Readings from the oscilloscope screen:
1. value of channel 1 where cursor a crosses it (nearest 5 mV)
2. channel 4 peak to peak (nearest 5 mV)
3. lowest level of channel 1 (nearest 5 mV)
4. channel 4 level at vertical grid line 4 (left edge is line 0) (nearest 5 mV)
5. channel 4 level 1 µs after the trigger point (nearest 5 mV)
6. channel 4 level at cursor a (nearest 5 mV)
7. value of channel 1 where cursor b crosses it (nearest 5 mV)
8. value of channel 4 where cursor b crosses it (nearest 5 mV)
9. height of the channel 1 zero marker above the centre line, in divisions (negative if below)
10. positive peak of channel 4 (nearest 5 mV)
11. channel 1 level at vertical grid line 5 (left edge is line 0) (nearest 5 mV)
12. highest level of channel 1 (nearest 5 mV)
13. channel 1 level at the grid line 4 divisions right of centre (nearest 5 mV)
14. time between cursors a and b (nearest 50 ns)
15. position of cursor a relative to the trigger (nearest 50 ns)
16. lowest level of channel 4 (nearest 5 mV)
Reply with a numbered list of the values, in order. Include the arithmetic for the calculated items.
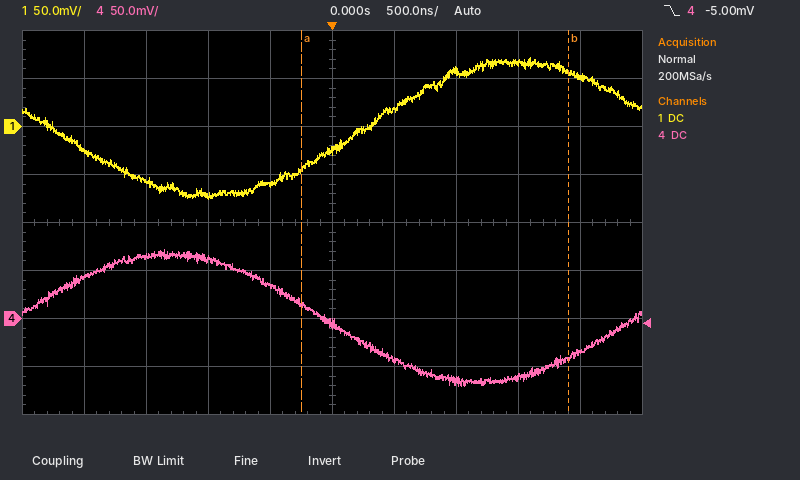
1. -45 mV
2. 70 mV − (-70 mV) = 140 mV
3. -75 mV
4. 35 mV
5. -65 mV
6. 15 mV
7. 55 mV
8. -40 mV
9. +2.0 div
10. 70 mV
11. -25 mV
12. 70 mV
13. 50 mV
14. 2.15 µs
15. -250 ns
16. -70 mV
